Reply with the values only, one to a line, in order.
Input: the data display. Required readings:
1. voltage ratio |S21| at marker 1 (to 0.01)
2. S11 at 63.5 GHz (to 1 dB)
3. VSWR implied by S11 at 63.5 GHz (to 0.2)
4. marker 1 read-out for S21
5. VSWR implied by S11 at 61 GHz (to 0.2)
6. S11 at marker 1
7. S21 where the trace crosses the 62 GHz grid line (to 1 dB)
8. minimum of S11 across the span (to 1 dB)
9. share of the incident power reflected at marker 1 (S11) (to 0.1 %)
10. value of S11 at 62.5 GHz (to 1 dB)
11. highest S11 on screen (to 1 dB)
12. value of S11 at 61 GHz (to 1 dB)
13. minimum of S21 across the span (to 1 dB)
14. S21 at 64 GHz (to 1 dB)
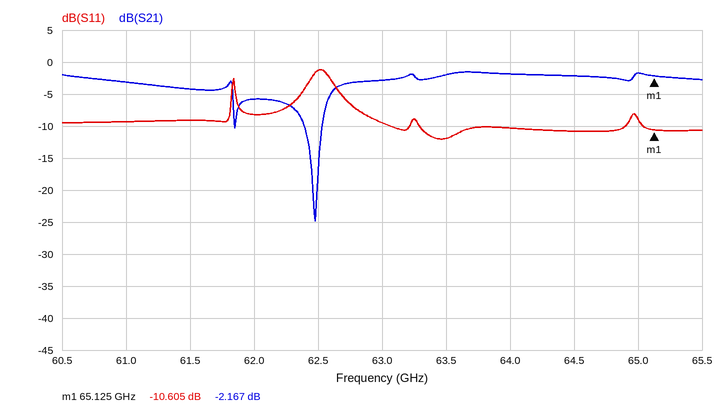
0.78
-12 dB
1.6
-2.167 dB
2.0
-10.605 dB
-6 dB
-12 dB
8.7 %
-1 dB
-1 dB
-9 dB
-25 dB
-2 dB
